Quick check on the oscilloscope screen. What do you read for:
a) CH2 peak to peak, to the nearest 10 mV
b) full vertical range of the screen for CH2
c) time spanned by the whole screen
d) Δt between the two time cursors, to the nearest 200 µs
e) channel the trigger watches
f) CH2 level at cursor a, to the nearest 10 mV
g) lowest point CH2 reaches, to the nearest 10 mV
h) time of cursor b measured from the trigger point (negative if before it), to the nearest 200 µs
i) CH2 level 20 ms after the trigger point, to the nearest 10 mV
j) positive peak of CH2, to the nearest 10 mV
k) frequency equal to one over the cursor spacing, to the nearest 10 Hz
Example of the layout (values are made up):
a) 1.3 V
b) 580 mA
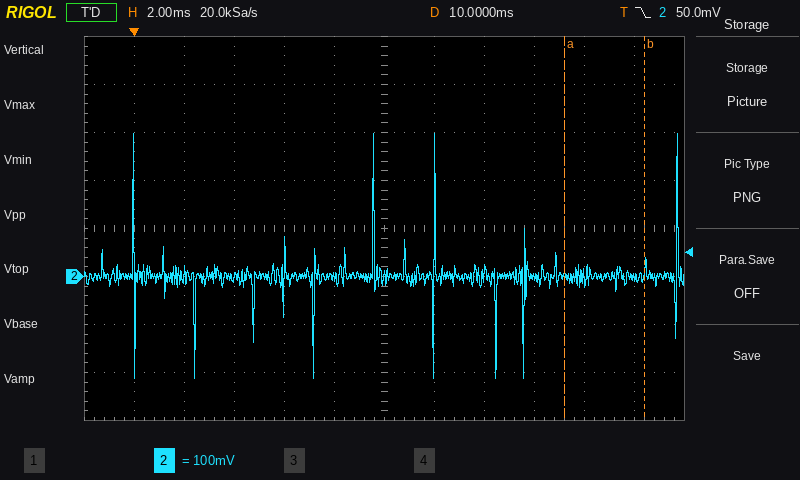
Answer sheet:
a) 510 mV
b) 800 mV
c) 24 ms
d) 3.2 ms
e) CH2
f) 0 mV
g) -210 mV
h) +20.4 ms
i) 0 mV
j) 300 mV
k) 310 Hz
